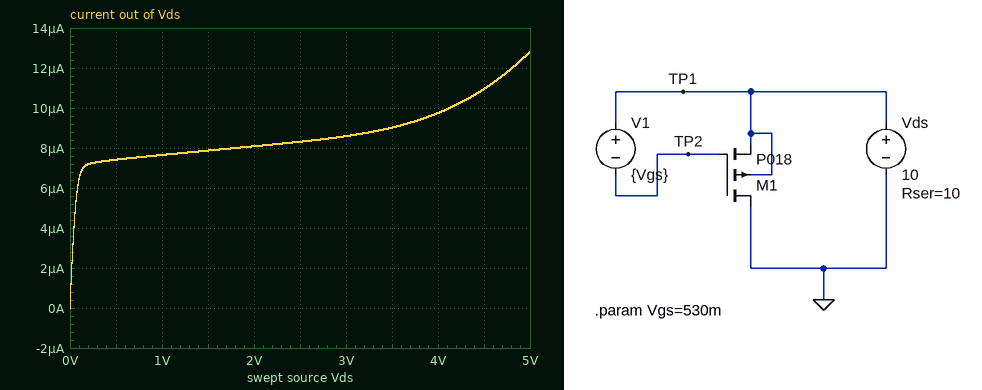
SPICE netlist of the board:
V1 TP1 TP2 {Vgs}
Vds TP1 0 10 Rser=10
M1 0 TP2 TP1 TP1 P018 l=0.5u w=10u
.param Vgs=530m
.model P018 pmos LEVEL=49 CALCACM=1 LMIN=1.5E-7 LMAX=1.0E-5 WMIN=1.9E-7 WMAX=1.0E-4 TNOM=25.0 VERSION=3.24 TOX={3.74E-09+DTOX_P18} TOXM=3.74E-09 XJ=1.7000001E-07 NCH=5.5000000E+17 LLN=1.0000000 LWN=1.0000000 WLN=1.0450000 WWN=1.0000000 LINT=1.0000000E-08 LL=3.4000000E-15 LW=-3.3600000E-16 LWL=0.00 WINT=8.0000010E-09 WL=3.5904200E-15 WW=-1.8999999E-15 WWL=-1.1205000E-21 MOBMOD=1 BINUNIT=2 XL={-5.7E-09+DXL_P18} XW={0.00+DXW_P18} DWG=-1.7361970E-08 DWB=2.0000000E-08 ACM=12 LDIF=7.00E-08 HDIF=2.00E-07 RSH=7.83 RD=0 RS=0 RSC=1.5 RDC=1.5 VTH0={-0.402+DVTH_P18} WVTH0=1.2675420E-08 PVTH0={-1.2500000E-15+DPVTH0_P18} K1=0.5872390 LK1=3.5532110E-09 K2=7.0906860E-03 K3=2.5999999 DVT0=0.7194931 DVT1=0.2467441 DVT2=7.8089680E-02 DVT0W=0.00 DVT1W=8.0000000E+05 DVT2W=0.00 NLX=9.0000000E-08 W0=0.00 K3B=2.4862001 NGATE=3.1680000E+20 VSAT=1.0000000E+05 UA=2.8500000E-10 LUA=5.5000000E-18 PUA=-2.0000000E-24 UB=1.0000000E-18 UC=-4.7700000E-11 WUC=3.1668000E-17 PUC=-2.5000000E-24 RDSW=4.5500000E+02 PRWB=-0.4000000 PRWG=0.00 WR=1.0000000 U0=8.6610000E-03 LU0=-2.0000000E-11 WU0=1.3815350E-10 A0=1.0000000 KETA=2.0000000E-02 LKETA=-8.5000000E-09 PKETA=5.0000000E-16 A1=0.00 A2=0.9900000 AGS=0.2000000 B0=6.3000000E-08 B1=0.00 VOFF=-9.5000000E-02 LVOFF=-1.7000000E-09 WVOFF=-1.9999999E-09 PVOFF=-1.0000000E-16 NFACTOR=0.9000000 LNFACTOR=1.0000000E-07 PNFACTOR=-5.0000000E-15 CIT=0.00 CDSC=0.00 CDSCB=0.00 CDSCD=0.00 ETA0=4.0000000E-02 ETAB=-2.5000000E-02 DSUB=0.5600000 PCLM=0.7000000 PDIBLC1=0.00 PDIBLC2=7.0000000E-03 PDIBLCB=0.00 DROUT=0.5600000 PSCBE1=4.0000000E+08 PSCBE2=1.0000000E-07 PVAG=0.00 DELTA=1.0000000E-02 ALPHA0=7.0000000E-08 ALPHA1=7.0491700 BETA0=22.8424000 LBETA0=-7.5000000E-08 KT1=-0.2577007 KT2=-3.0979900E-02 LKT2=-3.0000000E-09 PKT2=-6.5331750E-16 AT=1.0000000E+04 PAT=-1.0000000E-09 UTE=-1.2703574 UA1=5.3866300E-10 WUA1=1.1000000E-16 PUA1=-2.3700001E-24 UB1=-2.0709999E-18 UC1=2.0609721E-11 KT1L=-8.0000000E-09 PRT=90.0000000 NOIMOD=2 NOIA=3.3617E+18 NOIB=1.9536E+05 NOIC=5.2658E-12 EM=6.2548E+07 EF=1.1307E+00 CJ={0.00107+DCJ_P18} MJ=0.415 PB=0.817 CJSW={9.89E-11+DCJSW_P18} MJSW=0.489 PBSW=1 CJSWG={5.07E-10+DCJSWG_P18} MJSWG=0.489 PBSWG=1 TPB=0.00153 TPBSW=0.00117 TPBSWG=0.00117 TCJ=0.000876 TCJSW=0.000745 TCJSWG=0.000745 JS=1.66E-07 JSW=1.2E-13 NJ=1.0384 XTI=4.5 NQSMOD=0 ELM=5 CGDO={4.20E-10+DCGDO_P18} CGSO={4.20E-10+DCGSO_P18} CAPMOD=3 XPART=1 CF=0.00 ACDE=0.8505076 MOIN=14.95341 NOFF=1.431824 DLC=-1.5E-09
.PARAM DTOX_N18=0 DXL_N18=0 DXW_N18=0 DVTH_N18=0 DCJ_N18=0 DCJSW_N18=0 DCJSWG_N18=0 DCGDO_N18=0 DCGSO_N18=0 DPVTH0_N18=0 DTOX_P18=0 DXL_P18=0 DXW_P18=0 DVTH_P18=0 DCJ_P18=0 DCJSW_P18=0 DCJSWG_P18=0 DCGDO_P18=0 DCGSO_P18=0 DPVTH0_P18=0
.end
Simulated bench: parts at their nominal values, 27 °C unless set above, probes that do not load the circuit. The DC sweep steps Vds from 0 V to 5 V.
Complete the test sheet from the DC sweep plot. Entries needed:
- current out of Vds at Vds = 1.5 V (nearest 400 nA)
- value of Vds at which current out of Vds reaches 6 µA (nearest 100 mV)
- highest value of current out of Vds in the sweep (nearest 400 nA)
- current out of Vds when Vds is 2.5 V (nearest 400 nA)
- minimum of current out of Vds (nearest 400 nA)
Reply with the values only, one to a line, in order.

8.0 µA
100 mV
12.8 µA
8.4 µA
0 A
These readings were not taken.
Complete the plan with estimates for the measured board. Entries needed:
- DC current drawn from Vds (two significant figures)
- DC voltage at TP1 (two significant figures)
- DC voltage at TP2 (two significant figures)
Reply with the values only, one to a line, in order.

98 µA
10 V
9.5 V
